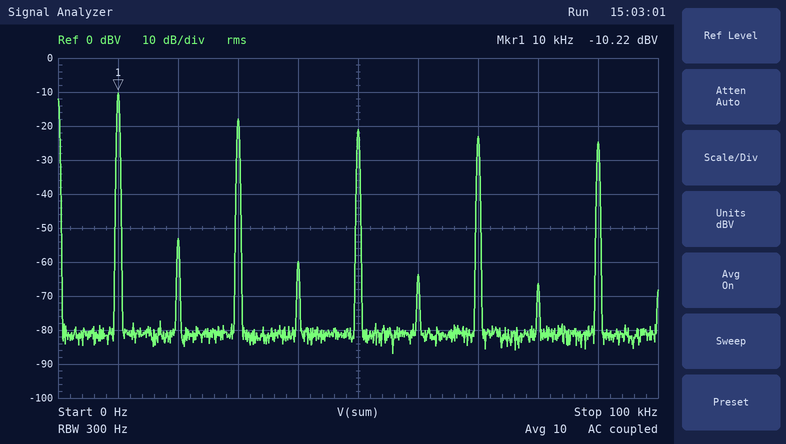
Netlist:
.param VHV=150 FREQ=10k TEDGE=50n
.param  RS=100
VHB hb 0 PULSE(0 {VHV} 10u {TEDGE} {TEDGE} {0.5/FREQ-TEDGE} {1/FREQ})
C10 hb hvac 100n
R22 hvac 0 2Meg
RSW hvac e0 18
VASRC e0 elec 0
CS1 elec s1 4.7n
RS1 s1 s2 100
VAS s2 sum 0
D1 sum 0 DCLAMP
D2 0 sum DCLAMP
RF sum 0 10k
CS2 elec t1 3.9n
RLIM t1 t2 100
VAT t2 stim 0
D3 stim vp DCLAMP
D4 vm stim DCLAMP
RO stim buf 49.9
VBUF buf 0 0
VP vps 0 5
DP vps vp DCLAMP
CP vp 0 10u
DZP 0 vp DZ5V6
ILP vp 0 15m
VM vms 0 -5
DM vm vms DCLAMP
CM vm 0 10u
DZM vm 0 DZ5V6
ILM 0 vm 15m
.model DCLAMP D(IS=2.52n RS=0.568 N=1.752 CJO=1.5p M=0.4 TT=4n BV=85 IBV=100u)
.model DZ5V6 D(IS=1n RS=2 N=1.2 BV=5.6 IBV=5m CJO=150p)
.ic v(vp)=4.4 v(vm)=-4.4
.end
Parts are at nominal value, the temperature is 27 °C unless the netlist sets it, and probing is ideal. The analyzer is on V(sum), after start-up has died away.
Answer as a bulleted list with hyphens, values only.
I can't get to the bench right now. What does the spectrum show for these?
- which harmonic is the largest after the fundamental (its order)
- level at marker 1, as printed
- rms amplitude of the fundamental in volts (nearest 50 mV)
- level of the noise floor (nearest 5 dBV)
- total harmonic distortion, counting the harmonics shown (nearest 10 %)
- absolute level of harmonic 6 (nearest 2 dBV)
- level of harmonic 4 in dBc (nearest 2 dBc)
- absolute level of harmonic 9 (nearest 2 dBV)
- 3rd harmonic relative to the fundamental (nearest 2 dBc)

- 3
- -10.22 dBV
- 300 mV
- -80 dBV
- 60 %
- -64 dBV
- -50 dBc
- -24 dBV
- -8 dBc
